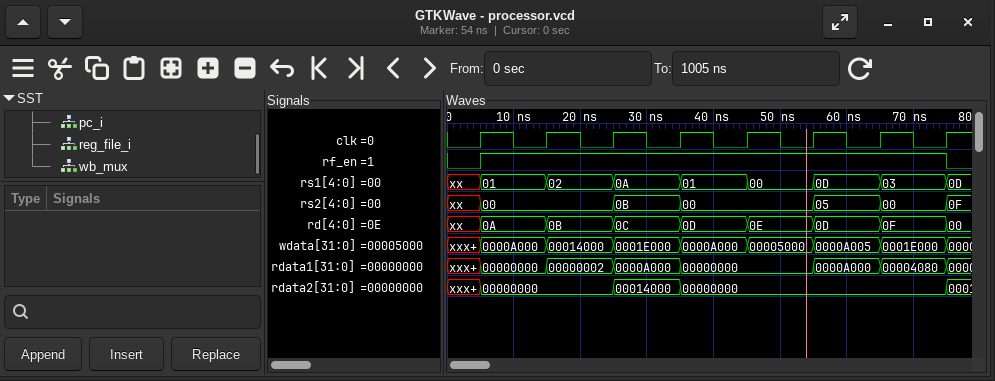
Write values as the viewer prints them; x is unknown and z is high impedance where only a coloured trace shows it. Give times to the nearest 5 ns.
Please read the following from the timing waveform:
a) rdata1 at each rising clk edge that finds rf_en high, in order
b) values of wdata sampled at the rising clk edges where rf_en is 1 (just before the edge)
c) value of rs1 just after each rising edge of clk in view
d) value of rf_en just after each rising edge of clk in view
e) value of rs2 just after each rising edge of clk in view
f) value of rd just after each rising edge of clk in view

00000000, 00000002, 0000A000, 00000000, 00000000, 0000A000, 00004080
0000A000, 00014000, 0001E000, 0000A000, 00005000, 0000A005, 0001E000
01, 02, 0A, 01, 00, 0D, 03, 0D
1 1 1 1 1 1 1 0
00, 00, 0B, 00, 00, 05, 00, 0F
0A, 0B, 0C, 0D, 0E, 0D, 0F, 00
